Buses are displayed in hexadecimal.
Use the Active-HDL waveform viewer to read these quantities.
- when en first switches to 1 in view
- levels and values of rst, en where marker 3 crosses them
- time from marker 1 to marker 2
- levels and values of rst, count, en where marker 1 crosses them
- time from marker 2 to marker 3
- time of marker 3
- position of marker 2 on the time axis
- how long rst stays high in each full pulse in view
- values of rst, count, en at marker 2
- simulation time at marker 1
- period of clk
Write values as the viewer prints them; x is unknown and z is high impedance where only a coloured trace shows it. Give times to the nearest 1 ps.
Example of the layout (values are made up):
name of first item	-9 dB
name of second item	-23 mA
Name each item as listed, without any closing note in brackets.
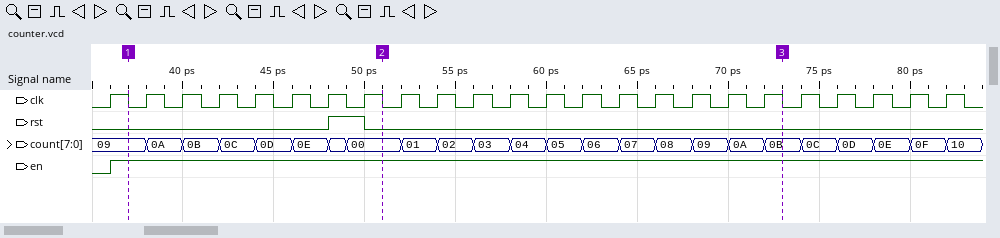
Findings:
when en first switches to 1 in view	36 ps
levels and values of rst, en where marker 3 crosses them	rst=0, en=1
time from marker 1 to marker 2	14 ps
levels and values of rst, count, en where marker 1 crosses them	rst=0, count=09, en=1
time from marker 2 to marker 3	22 ps
time of marker 3	73 ps
position of marker 2 on the time axis	51 ps
how long rst stays high in each full pulse in view	2 ps
values of rst, count, en at marker 2	rst=0, count=00, en=1
simulation time at marker 1	37 ps
period of clk	2 ps
